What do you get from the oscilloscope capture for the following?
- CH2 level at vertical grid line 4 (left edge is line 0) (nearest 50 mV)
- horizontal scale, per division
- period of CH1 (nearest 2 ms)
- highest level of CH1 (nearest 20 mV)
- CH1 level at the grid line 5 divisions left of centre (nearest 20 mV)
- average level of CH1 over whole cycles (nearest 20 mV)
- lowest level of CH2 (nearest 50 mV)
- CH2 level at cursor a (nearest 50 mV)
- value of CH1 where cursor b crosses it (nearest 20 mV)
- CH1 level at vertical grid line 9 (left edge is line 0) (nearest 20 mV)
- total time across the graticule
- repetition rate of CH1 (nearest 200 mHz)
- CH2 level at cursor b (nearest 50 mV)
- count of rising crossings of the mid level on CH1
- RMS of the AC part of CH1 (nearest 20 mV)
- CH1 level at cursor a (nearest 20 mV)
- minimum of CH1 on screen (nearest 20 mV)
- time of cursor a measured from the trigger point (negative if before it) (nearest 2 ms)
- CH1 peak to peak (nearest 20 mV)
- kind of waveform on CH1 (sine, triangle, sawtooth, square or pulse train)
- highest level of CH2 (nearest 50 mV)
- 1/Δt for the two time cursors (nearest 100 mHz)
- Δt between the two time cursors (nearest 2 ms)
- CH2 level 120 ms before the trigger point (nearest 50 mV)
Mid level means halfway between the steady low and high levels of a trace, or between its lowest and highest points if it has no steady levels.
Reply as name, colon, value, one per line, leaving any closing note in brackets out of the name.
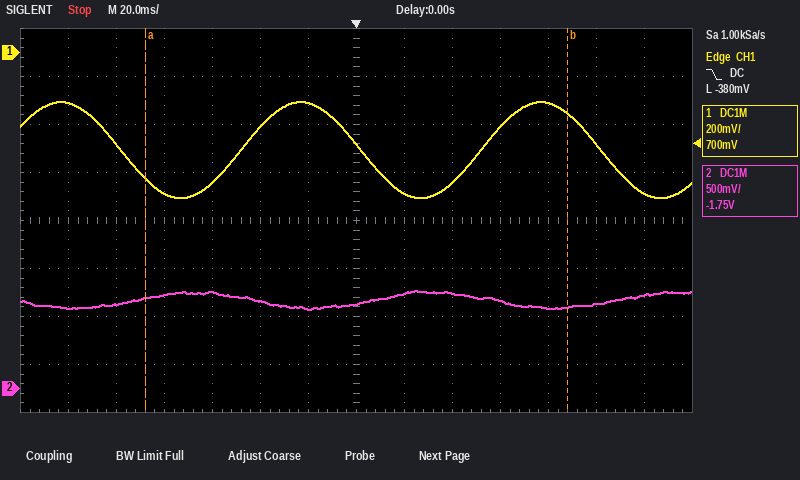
CH2 level at vertical grid line 4 (left edge is line 0): 1.00 V
horizontal scale, per division: 20 ms
period of CH1: 100 ms
highest level of CH1: -200 mV
CH1 level at the grid line 5 divisions left of centre: -380 mV
average level of CH1 over whole cycles: -400 mV
lowest level of CH2: 800 mV
CH2 level at cursor a: 950 mV
value of CH1 where cursor b crosses it: -260 mV
CH1 level at vertical grid line 9 (left edge is line 0): -540 mV
total time across the graticule: 280 ms
repetition rate of CH1: 10.0 Hz
CH2 level at cursor b: 850 mV
count of rising crossings of the mid level on CH1: 2
RMS of the AC part of CH1: 140 mV
CH1 level at cursor a: -520 mV
minimum of CH1 on screen: -600 mV
time of cursor a measured from the trigger point (negative if before it): -88 ms
CH1 peak to peak: 400 mV
kind of waveform on CH1: sine
highest level of CH2: 1.00 V
1/Δt for the two time cursors: 5.7 Hz
Δt between the two time cursors: 176 ms
CH2 level 120 ms before the trigger point: 850 mV
